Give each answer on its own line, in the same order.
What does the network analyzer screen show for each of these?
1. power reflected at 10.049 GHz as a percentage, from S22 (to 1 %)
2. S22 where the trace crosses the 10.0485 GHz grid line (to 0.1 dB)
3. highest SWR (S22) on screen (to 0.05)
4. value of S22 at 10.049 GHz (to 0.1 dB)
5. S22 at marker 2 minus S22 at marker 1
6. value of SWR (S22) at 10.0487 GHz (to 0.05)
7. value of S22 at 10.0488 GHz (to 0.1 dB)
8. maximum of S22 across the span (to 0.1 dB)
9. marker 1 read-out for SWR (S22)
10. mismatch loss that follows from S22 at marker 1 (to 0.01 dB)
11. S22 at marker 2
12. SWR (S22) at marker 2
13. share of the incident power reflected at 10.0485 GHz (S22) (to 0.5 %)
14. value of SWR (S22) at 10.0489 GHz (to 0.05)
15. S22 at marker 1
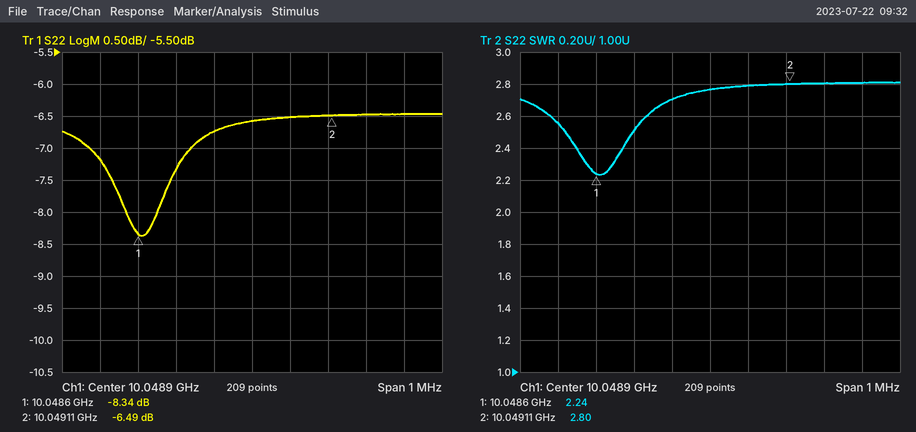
22 %
-7.2 dB
2.80
-6.5 dB
1.85 dB
2.50
-6.7 dB
-6.5 dB
2.24
0.69 dB
-6.49 dB
2.80
19.0 %
2.75
-8.34 dB
